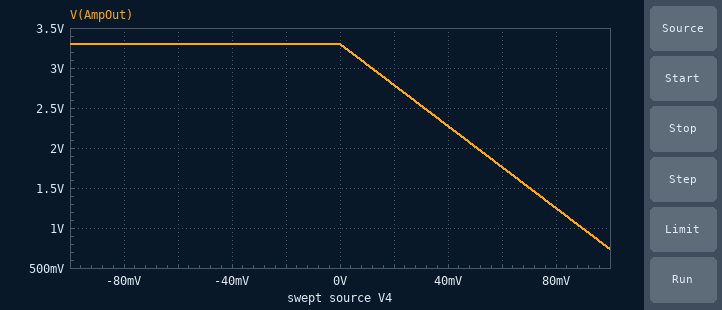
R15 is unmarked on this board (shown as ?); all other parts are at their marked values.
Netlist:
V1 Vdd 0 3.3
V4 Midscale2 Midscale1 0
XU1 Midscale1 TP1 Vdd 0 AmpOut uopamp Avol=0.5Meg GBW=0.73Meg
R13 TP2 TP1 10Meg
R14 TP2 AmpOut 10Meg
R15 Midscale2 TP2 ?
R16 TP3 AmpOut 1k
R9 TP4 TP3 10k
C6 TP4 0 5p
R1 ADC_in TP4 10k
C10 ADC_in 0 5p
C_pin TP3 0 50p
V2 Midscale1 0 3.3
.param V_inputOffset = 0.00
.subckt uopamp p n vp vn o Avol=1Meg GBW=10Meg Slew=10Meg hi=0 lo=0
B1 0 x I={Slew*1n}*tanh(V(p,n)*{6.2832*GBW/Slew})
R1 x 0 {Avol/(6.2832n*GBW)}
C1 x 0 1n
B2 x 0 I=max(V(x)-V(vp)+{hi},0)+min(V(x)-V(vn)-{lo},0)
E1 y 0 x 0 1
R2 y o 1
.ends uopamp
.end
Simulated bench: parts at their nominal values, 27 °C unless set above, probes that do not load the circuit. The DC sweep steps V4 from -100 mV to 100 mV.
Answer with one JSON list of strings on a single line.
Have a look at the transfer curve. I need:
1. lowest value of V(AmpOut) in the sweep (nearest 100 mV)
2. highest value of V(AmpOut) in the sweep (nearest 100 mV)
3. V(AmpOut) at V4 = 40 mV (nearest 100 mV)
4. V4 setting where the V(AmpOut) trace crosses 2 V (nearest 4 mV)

["700 mV", "3.3 V", "2.3 V", "52 mV"]
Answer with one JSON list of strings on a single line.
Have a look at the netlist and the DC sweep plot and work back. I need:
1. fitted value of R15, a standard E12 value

["390 kΩ"]
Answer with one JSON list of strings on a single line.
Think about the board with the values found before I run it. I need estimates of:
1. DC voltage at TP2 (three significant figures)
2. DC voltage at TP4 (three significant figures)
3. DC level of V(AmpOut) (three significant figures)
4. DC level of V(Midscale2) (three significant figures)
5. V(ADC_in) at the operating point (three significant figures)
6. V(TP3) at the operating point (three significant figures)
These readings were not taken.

["3.30 V", "3.30 V", "3.30 V", "3.30 V", "3.30 V", "3.30 V"]
